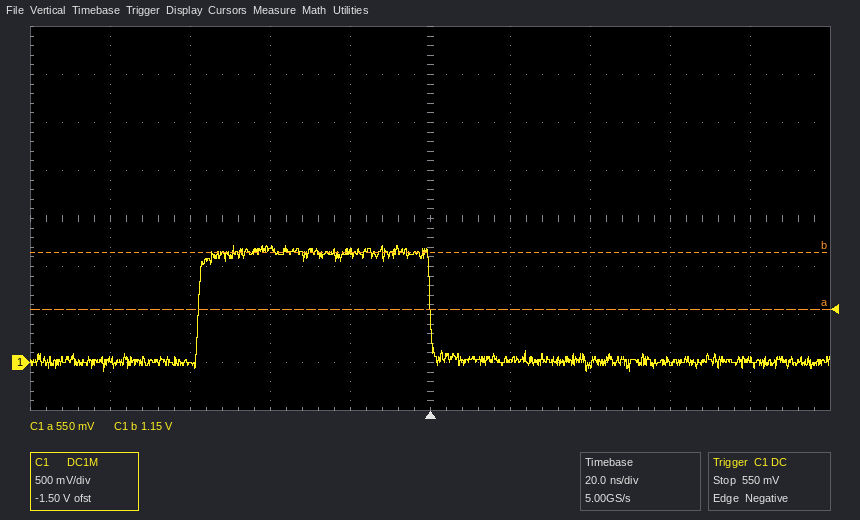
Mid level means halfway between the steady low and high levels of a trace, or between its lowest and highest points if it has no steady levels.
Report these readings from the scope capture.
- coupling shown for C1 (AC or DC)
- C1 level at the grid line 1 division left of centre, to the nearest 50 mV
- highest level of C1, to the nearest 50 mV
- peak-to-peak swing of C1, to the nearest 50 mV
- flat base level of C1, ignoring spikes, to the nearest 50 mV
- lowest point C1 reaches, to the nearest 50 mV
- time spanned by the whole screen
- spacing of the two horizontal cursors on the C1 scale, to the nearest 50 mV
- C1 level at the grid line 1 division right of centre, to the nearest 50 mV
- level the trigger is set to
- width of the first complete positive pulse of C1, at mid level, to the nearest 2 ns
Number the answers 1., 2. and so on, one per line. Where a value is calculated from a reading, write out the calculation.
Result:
1. DC
2. 1.15 V
3. 1.20 V
4. 1.20 V − (-100 mV) = 1.30 V
5. 0 mV
6. -100 mV
7. 200 ns
8. 600 mV
9. 50 mV
10. 550 mV
11. 58 ns
